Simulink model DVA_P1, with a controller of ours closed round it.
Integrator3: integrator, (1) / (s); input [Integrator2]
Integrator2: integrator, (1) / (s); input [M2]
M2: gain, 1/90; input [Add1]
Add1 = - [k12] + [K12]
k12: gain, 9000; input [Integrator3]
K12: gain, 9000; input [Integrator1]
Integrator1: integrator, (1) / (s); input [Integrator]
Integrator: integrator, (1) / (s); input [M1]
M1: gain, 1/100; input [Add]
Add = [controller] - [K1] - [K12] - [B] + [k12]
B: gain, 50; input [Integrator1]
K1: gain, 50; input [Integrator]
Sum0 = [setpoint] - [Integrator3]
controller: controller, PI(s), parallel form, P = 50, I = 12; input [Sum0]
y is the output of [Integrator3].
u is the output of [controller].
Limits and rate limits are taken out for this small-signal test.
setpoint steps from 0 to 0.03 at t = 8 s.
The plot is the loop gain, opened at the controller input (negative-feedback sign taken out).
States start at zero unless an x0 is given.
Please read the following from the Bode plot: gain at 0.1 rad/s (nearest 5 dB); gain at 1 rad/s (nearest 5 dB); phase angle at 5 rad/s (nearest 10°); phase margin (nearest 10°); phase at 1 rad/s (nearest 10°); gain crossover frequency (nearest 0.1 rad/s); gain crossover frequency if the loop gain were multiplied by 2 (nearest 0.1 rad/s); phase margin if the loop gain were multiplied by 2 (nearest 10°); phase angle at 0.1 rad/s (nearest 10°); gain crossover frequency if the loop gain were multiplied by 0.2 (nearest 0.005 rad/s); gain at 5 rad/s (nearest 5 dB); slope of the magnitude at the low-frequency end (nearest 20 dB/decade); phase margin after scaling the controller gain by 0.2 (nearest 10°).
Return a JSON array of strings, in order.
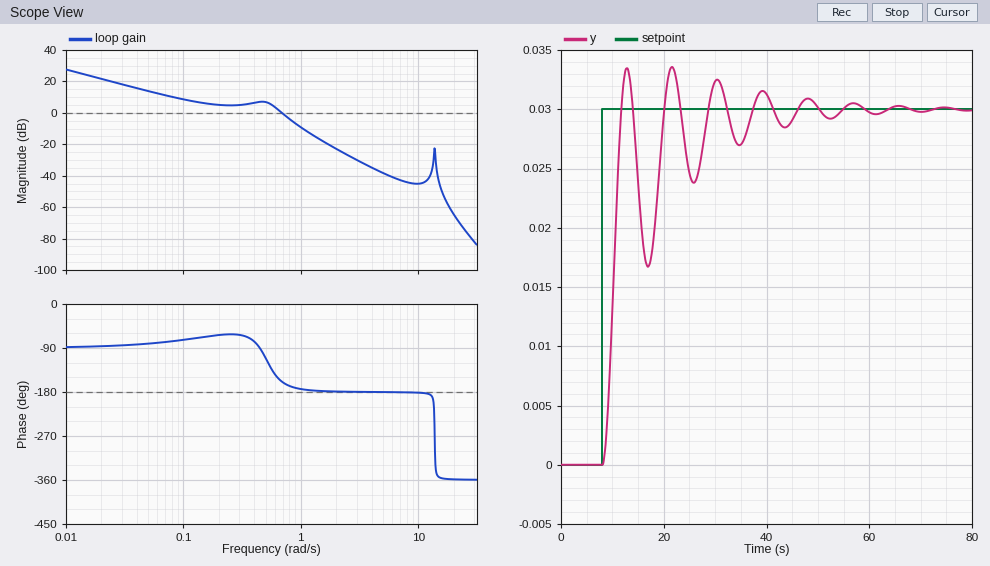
["10 dB", "-10 dB", "-180°", "20°", "-170°", "0.7 rad/s", "0.9 rad/s", "10°", "-70°", "0.050 rad/s", "-40 dB", "-20 dB/decade", "100°"]
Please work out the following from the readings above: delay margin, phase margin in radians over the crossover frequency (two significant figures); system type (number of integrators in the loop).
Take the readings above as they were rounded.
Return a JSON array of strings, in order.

["0.50 s", "1"]
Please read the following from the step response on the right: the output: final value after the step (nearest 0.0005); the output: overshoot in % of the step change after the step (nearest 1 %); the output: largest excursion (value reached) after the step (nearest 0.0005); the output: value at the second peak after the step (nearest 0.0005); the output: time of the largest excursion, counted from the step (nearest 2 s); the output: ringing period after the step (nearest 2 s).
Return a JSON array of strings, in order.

["0.0300", "12 %", "0.0335", "0.0335", "14 s", "8 s"]
